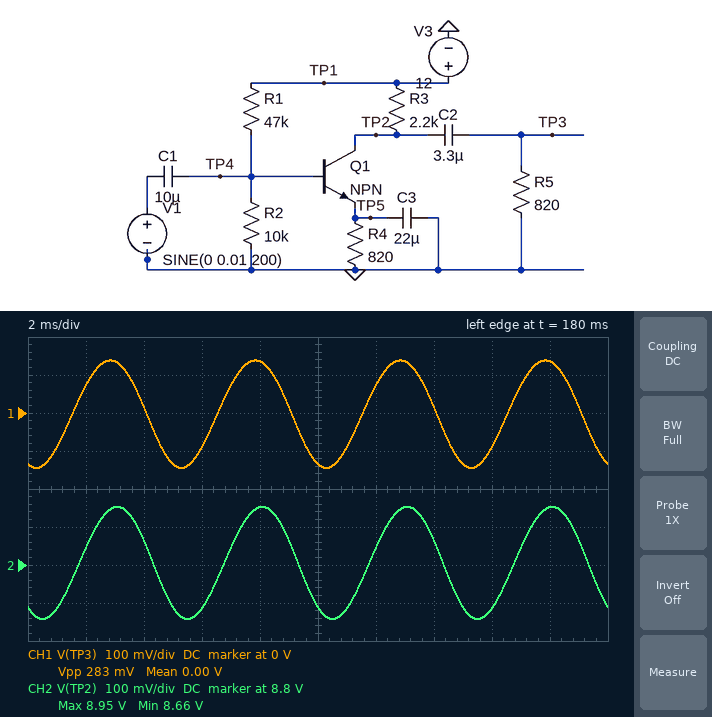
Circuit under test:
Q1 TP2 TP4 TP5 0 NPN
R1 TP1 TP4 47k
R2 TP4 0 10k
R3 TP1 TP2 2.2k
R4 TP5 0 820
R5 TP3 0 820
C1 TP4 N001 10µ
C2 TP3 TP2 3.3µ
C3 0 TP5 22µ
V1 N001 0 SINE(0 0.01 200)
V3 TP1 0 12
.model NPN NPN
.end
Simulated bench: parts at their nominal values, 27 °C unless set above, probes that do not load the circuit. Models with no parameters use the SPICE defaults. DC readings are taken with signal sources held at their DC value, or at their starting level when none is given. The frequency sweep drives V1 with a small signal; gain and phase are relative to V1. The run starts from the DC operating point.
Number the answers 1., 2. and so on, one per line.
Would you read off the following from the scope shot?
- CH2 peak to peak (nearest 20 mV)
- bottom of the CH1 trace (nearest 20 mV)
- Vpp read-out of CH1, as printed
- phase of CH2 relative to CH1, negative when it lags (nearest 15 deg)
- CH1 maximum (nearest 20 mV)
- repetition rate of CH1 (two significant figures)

1. 300 mV
2. -140 mV
3. 283 mV
4. -15 deg
5. 140 mV
6. 200 Hz
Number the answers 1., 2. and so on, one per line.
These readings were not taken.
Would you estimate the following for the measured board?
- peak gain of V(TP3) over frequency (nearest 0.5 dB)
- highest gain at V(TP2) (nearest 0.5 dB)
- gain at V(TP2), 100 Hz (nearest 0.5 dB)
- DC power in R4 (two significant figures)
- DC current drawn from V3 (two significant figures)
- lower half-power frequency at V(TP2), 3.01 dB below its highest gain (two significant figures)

1. 30.5 dB
2. 30.5 dB
3. 19.0 dB
4. 1.8 mW
5. 1.7 mA
6. 420 Hz
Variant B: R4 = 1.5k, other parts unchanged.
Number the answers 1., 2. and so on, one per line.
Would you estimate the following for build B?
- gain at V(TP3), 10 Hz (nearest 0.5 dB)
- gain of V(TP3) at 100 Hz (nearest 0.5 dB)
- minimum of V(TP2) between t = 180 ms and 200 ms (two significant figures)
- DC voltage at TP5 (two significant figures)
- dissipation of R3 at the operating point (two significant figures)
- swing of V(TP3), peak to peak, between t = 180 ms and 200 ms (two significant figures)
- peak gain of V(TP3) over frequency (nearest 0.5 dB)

1. -7.0 dB
2. 17.0 dB
3. 10 V
4. 1.3 V
5. 1.5 mW
6. 240 mV
7. 25.5 dB
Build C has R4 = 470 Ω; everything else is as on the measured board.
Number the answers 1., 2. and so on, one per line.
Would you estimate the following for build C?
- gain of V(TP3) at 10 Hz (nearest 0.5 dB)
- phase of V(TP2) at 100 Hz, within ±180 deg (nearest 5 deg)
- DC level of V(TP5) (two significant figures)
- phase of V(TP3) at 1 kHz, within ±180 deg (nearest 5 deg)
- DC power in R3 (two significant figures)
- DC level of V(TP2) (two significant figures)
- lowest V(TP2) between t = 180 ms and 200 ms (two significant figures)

1. -2.5 dB
2. -125 deg
3. 1.1 V
4. -145 deg
5. 12 mW
6. 6.8 V
7. 6.7 V
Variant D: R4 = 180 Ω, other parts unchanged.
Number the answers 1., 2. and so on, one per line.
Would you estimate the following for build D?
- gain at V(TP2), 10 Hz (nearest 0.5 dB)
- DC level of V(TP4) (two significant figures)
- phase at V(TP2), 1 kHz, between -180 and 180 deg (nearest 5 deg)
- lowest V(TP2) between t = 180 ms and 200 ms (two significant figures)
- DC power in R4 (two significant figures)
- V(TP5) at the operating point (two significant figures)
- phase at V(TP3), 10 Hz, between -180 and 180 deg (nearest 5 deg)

1. 20.0 dB
2. 1.7 V
3. -130 deg
4. 1.1 V
5. 4.4 mW
6. 890 mV
7. -95 deg
